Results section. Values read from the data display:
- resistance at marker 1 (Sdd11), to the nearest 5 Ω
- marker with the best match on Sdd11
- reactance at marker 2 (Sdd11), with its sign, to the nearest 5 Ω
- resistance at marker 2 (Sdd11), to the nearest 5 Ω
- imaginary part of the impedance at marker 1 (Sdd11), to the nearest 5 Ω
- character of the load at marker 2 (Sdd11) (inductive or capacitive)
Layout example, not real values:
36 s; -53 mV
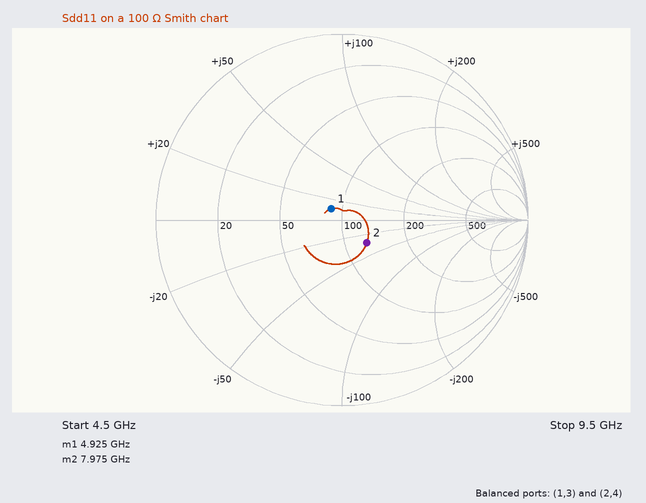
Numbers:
90 Ω; marker 1; -30 Ω; 125 Ω; +10 Ω; capacitive
